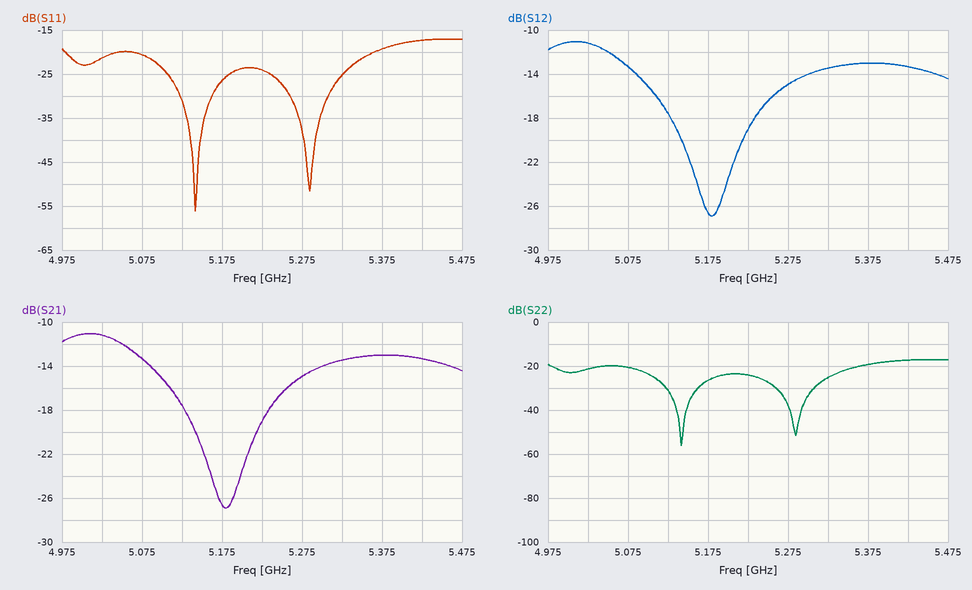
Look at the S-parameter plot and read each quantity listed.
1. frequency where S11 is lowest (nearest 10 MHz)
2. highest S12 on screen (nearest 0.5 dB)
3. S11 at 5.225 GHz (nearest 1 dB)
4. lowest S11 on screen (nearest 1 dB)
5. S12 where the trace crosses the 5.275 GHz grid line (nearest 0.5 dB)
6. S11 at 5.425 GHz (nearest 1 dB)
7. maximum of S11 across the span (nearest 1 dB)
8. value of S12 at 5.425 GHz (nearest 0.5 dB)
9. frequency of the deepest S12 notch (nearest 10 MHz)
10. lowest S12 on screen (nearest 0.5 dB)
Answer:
5.14 GHz
-11.0 dB
-24 dB
-56 dB
-15.0 dB
-17 dB
-17 dB
-13.5 dB
5.18 GHz
-27.0 dB
